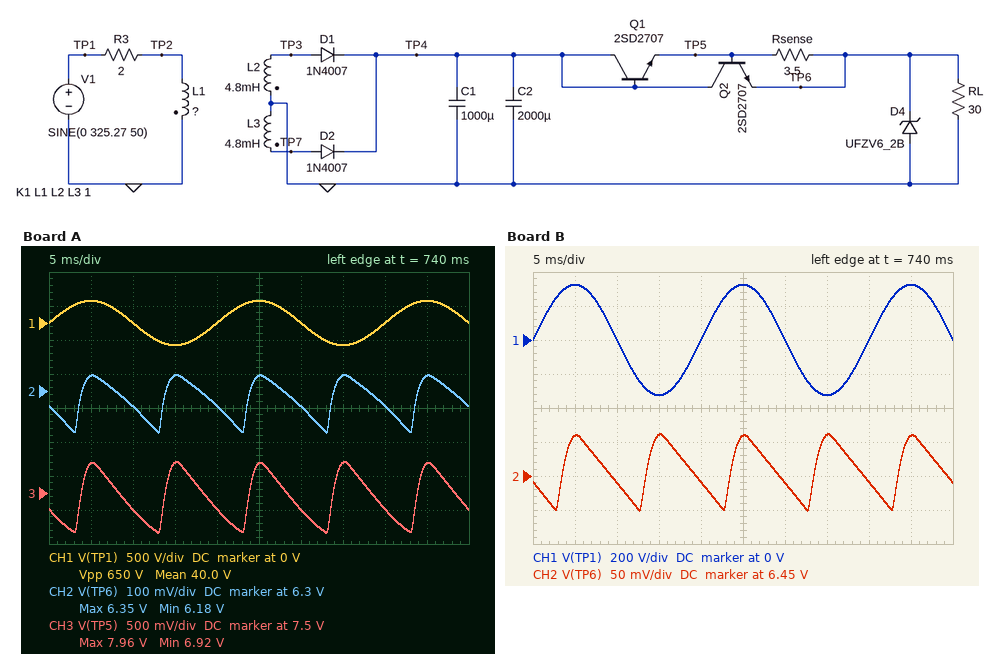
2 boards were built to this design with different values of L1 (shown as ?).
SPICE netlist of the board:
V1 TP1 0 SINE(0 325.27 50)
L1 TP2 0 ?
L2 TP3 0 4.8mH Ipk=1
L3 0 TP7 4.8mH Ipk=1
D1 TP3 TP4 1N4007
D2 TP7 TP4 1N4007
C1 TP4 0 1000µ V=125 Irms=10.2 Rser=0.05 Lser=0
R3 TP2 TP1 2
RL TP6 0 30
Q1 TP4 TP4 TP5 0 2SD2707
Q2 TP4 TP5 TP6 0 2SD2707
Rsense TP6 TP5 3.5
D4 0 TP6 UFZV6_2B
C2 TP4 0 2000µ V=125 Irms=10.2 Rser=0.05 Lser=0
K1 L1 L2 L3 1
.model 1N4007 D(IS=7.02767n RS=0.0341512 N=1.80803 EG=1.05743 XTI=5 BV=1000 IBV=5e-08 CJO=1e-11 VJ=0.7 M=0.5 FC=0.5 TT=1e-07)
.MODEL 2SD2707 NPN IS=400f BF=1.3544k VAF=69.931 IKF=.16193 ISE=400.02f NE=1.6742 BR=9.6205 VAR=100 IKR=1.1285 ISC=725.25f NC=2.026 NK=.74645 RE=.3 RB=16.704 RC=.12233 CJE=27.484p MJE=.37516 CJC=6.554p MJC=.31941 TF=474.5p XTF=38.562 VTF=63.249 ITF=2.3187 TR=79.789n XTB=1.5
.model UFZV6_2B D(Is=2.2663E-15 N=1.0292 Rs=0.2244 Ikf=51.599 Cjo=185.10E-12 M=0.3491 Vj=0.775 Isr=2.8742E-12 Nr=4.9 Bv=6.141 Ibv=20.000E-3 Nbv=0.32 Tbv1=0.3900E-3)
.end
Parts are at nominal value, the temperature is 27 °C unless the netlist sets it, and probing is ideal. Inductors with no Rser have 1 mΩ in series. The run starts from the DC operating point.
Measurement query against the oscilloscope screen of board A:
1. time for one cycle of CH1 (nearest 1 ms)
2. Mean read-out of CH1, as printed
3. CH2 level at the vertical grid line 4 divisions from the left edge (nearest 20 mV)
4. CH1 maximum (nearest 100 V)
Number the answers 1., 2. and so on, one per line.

1. 20 ms
2. 40.0 V
3. 6.26 V
4. 300 V
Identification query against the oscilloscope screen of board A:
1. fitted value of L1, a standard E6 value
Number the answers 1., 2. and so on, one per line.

1. 4.7 H
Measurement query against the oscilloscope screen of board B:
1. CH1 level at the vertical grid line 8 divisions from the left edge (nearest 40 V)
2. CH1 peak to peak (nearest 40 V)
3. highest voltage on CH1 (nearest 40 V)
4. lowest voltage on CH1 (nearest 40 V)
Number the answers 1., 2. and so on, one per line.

1. 0 V
2. 640 V
3. 320 V
4. -320 V
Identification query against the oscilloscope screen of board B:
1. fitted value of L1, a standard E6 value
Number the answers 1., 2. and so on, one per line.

1. 2.2 H
